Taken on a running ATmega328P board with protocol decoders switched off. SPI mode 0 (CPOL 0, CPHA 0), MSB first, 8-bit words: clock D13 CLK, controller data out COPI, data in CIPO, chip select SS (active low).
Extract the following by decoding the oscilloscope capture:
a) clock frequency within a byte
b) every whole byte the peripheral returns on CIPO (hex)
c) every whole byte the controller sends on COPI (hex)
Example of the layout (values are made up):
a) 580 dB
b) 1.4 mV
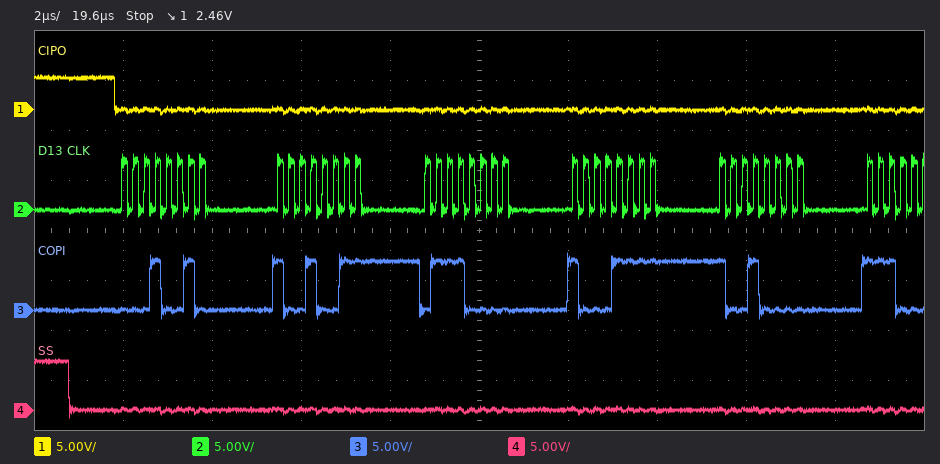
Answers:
a) 4 MHz
b) 00 00 00 00 00
c) 12 93 70 8F 90
